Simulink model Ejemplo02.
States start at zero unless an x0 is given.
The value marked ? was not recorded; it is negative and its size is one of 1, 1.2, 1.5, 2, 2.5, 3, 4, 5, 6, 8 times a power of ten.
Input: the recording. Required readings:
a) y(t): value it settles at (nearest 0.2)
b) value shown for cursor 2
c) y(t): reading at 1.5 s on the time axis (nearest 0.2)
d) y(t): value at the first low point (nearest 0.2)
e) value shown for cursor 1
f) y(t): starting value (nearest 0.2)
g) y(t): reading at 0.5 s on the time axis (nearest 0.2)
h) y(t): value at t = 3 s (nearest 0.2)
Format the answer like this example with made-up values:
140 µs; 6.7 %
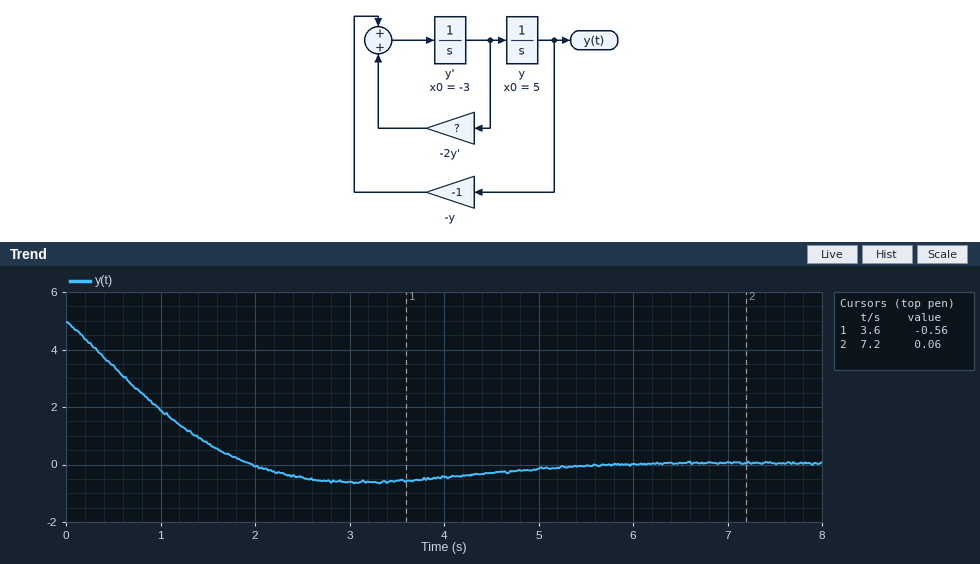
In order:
0.0; 0.06; 0.8; -0.6; -0.56; 5.0; 3.4; -0.6
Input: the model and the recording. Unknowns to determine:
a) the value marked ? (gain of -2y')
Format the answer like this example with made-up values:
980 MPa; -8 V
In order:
-1.2
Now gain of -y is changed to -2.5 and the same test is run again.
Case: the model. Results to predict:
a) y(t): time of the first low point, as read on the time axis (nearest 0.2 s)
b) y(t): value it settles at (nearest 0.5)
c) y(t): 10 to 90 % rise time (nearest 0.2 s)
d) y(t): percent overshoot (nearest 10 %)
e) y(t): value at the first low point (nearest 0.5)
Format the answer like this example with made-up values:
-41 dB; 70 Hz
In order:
1.8 s; 0.0; 0.8 s; 30 %; -1.5
